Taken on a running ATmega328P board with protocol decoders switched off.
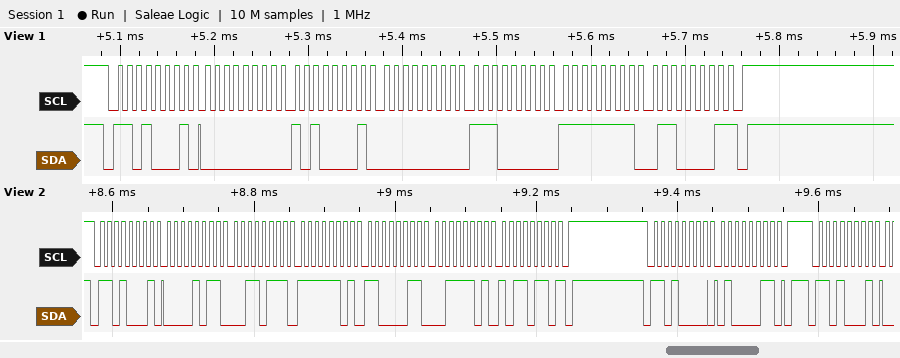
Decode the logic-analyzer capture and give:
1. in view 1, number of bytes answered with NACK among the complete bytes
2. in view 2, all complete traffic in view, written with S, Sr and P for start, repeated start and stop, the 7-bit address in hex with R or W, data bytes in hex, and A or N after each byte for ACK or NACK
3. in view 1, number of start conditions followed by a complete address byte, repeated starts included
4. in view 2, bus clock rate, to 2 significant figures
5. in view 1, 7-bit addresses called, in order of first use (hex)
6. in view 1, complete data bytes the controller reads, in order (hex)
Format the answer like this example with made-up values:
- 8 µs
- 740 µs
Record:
- 1
- S 68R A 0B A 37 A FD A C3 A 3D A B6 N P S 68W A 43 A P S 68R A
- 1
- 100 kHz
- 0x68
- 00 A1 00 E0 FF 61
